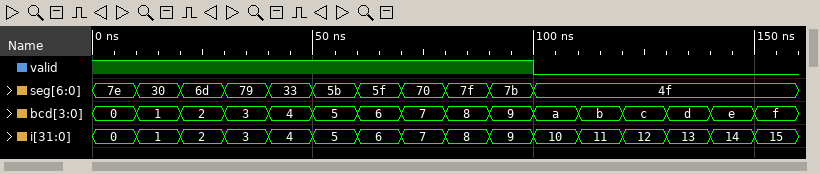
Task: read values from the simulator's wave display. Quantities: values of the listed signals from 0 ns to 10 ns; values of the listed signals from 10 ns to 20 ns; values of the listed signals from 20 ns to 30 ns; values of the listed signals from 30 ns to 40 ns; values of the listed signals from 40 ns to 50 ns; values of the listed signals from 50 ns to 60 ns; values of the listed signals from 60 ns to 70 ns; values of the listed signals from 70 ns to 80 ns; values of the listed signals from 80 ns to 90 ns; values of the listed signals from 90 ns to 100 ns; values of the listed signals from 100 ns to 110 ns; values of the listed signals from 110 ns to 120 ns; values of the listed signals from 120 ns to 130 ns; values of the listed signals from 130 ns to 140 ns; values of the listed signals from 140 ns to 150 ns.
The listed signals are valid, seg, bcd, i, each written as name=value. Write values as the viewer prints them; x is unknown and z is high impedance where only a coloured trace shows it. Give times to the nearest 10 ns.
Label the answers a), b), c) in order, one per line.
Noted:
a) valid=1, seg=7e, bcd=0, i=0
b) valid=1, seg=30, bcd=1, i=1
c) valid=1, seg=6d, bcd=2, i=2
d) valid=1, seg=79, bcd=3, i=3
e) valid=1, seg=33, bcd=4, i=4
f) valid=1, seg=5b, bcd=5, i=5
g) valid=1, seg=5f, bcd=6, i=6
h) valid=1, seg=70, bcd=7, i=7
i) valid=1, seg=7f, bcd=8, i=8
j) valid=1, seg=7b, bcd=9, i=9
k) valid=0, seg=4f, bcd=a, i=10
l) valid=0, seg=4f, bcd=b, i=11
m) valid=0, seg=4f, bcd=c, i=12
n) valid=0, seg=4f, bcd=d, i=13
o) valid=0, seg=4f, bcd=e, i=14
